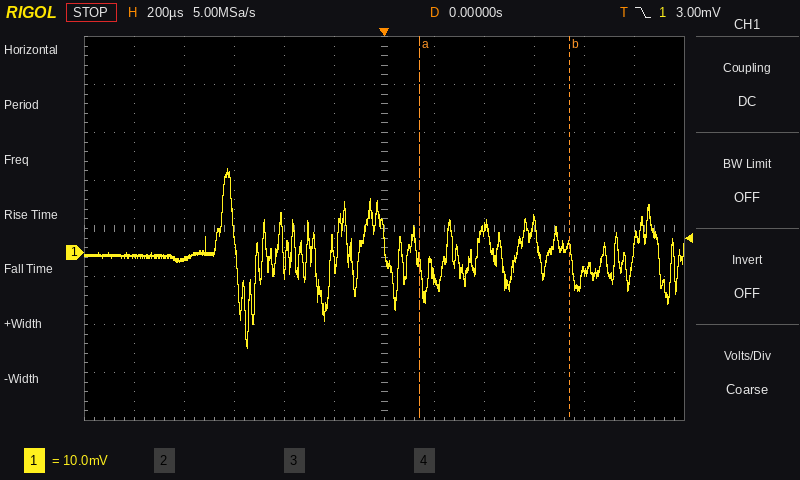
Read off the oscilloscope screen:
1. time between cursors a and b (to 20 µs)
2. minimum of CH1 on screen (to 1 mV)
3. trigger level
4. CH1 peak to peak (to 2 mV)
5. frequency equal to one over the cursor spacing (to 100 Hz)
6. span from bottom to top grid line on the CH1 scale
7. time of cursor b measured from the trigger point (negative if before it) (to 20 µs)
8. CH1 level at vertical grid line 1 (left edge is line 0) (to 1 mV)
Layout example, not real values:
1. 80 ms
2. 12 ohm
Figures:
1. 600 µs
2. -20 mV
3. 3.00 mV
4. 38 mV
5. 1.7 kHz
6. 80 mV
7. +740 µs
8. -1 mV
